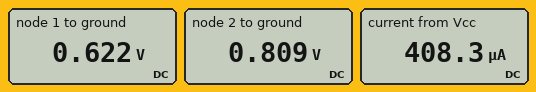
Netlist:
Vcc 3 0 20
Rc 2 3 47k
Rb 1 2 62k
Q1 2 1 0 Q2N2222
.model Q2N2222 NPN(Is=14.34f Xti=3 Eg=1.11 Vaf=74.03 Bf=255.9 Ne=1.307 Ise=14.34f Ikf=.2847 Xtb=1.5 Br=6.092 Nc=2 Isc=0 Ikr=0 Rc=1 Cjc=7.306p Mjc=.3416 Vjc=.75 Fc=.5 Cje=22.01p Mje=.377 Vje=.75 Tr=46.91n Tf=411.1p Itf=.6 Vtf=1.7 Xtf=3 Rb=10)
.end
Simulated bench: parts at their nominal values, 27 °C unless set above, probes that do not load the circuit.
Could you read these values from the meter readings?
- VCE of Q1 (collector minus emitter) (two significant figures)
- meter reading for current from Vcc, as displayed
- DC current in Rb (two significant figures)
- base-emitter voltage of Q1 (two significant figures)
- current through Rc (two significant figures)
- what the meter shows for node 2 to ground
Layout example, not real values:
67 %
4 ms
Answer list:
810 mV
408.3 µA
3.0 µA
620 mV
410 µA
0.809 V
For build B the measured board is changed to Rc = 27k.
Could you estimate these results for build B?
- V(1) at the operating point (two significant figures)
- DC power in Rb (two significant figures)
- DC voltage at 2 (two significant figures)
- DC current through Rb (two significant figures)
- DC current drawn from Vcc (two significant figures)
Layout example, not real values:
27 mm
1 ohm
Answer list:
640 mV
1.5 µW
940 mV
4.9 µA
710 µA
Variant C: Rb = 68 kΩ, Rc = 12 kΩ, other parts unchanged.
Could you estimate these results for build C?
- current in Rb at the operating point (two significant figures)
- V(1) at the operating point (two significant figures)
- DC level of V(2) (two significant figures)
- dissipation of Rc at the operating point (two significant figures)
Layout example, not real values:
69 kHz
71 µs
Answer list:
10 µA
660 mV
1.3 V
29 mW
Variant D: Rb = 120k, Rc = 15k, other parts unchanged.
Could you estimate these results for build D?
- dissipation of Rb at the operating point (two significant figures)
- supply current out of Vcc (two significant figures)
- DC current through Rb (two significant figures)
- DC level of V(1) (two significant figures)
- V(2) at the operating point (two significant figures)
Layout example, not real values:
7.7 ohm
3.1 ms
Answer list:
7.7 µW
1.2 mA
8.0 µA
650 mV
1.6 V
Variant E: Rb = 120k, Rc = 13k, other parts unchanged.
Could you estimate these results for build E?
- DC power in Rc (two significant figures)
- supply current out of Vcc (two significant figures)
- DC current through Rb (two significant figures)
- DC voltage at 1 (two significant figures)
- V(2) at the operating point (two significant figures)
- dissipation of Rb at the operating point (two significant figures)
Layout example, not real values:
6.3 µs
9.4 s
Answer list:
26 mW
1.4 mA
9.0 µA
650 mV
1.7 V
9.8 µW
